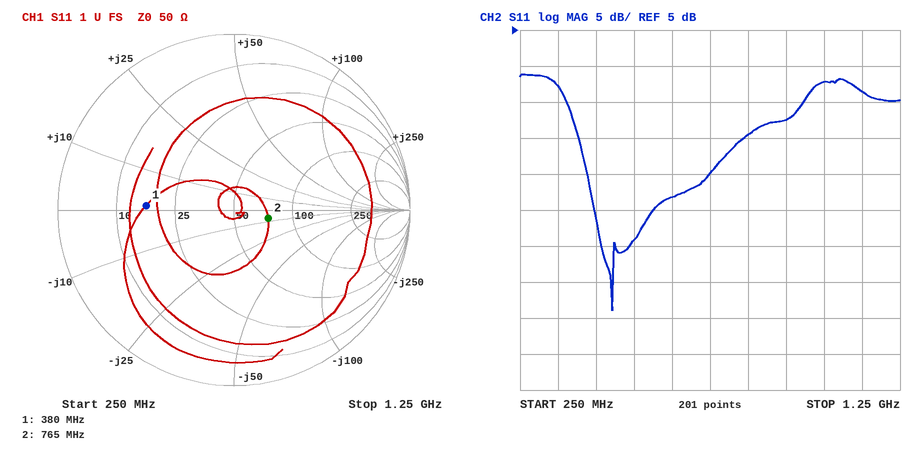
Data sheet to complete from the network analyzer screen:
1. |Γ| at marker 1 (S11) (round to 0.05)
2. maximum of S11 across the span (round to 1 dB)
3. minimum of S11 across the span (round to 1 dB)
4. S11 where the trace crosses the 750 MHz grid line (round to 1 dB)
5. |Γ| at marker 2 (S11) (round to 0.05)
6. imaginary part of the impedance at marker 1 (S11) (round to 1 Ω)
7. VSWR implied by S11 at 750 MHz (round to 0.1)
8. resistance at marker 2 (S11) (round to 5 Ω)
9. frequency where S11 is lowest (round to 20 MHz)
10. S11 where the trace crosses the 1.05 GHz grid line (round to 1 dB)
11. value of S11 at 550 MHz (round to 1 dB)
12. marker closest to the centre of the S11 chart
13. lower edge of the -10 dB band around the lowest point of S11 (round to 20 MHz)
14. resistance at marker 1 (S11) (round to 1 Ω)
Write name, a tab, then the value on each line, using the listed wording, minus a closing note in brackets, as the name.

|Γ| at marker 1 (S11)	0.50
maximum of S11 across the span	-1 dB
minimum of S11 across the span	-34 dB
S11 where the trace crosses the 750 MHz grid line	-15 dB
|Γ| at marker 2 (S11)	0.20
imaginary part of the impedance at marker 1 (S11)	+1 Ω
VSWR implied by S11 at 750 MHz	1.4
resistance at marker 2 (S11)	75 Ω
frequency where S11 is lowest	500 MHz
S11 where the trace crosses the 1.05 GHz grid line	-2 dB
value of S11 at 550 MHz	-24 dB
marker closest to the centre of the S11 chart	marker 2
lower edge of the -10 dB band around the lowest point of S11	400 MHz
resistance at marker 1 (S11)	17 Ω
